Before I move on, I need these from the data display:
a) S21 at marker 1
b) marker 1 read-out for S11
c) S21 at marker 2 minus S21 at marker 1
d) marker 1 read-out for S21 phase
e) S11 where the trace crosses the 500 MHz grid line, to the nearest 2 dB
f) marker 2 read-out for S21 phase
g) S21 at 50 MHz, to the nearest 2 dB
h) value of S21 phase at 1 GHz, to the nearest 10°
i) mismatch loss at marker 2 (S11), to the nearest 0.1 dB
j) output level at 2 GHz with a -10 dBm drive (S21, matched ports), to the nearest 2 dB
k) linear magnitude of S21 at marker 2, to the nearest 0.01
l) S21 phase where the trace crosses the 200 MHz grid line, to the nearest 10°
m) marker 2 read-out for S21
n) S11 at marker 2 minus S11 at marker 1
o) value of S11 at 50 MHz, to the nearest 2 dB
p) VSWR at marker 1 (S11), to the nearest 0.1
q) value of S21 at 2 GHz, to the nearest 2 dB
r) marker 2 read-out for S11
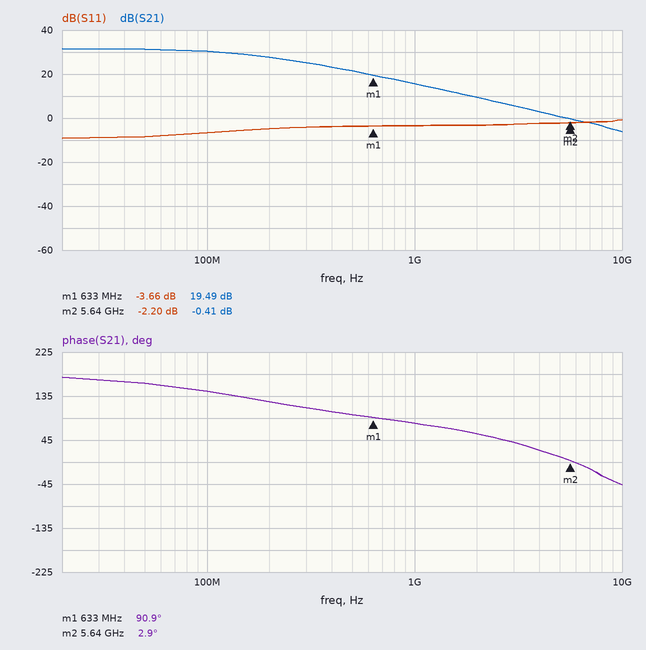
19.49 dB
-3.66 dB
-19.90 dB
90.9°
-4 dB
2.9°
32 dB
80°
4.0 dB
0 dBm
0.95
120°
-0.41 dB
1.46 dB
-8 dB
4.8
10 dB
-2.20 dB
